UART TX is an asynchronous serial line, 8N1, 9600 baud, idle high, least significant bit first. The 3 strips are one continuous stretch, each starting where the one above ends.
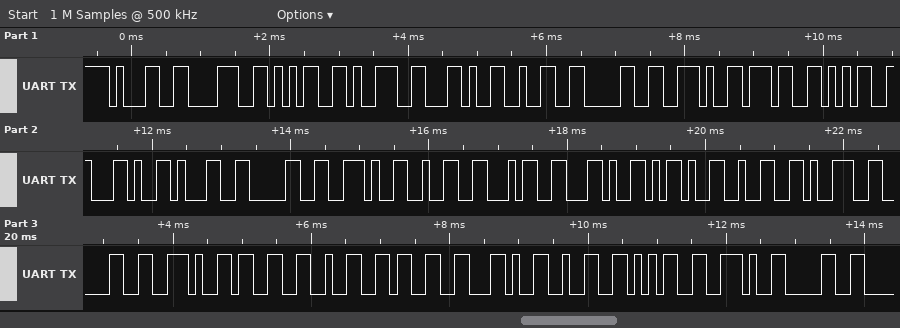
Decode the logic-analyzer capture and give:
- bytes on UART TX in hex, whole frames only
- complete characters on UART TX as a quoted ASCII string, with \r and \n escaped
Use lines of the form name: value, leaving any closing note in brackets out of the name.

bytes on UART TX in hex, whole frames only: 31 38 35 39 2C 32 30 2E 37 35 2C 31 30 2E 32 34 2C 2D 32 39 30 2E 33 32 33 2C 32 35 2E 30
complete characters on UART TX as a quoted ASCII string, with \r and \n escaped: "1859,20.75,10.24,-290.323,25.0"
